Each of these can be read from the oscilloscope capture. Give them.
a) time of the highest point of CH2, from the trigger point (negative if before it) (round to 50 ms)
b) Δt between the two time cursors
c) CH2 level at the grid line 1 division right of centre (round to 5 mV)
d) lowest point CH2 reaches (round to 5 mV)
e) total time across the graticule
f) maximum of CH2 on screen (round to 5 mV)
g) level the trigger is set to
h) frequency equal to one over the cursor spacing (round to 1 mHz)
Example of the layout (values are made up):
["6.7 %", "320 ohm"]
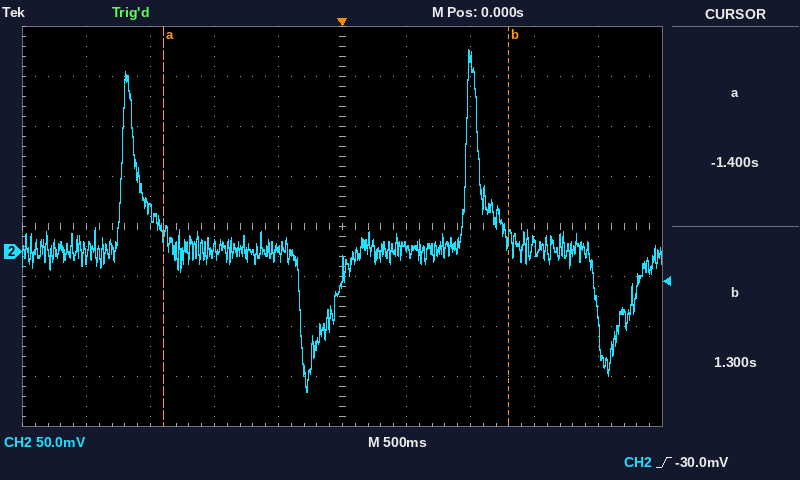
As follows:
["+1.00 s", "2.70 s", "5 mV", "-140 mV", "5 s", "200 mV", "-30.0 mV", "370 mHz"]
